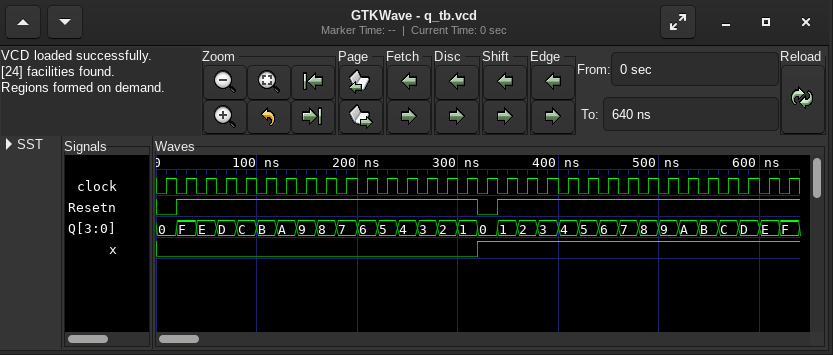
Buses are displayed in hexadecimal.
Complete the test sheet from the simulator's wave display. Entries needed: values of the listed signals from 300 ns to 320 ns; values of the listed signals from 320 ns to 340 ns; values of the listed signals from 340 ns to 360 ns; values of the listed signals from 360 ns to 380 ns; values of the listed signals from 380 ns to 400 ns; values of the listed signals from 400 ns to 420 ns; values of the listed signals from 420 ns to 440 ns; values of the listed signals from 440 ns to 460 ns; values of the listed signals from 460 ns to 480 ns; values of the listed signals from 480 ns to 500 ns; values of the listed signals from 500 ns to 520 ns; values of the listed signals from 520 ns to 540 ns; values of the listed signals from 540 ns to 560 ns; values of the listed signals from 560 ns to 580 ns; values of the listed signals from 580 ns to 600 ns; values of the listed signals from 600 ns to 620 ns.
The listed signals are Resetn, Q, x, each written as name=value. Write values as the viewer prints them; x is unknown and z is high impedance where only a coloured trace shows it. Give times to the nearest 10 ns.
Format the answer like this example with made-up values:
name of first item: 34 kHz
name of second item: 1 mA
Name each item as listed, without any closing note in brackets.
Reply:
values of the listed signals from 300 ns to 320 ns: Resetn=1, Q=1, x=0
values of the listed signals from 320 ns to 340 ns: Resetn=0, Q=0, x=1
values of the listed signals from 340 ns to 360 ns: Resetn=1, Q=1, x=1
values of the listed signals from 360 ns to 380 ns: Resetn=1, Q=2, x=1
values of the listed signals from 380 ns to 400 ns: Resetn=1, Q=3, x=1
values of the listed signals from 400 ns to 420 ns: Resetn=1, Q=4, x=1
values of the listed signals from 420 ns to 440 ns: Resetn=1, Q=5, x=1
values of the listed signals from 440 ns to 460 ns: Resetn=1, Q=6, x=1
values of the listed signals from 460 ns to 480 ns: Resetn=1, Q=7, x=1
values of the listed signals from 480 ns to 500 ns: Resetn=1, Q=8, x=1
values of the listed signals from 500 ns to 520 ns: Resetn=1, Q=9, x=1
values of the listed signals from 520 ns to 540 ns: Resetn=1, Q=A, x=1
values of the listed signals from 540 ns to 560 ns: Resetn=1, Q=B, x=1
values of the listed signals from 560 ns to 580 ns: Resetn=1, Q=C, x=1
values of the listed signals from 580 ns to 600 ns: Resetn=1, Q=D, x=1
values of the listed signals from 600 ns to 620 ns: Resetn=1, Q=E, x=1
